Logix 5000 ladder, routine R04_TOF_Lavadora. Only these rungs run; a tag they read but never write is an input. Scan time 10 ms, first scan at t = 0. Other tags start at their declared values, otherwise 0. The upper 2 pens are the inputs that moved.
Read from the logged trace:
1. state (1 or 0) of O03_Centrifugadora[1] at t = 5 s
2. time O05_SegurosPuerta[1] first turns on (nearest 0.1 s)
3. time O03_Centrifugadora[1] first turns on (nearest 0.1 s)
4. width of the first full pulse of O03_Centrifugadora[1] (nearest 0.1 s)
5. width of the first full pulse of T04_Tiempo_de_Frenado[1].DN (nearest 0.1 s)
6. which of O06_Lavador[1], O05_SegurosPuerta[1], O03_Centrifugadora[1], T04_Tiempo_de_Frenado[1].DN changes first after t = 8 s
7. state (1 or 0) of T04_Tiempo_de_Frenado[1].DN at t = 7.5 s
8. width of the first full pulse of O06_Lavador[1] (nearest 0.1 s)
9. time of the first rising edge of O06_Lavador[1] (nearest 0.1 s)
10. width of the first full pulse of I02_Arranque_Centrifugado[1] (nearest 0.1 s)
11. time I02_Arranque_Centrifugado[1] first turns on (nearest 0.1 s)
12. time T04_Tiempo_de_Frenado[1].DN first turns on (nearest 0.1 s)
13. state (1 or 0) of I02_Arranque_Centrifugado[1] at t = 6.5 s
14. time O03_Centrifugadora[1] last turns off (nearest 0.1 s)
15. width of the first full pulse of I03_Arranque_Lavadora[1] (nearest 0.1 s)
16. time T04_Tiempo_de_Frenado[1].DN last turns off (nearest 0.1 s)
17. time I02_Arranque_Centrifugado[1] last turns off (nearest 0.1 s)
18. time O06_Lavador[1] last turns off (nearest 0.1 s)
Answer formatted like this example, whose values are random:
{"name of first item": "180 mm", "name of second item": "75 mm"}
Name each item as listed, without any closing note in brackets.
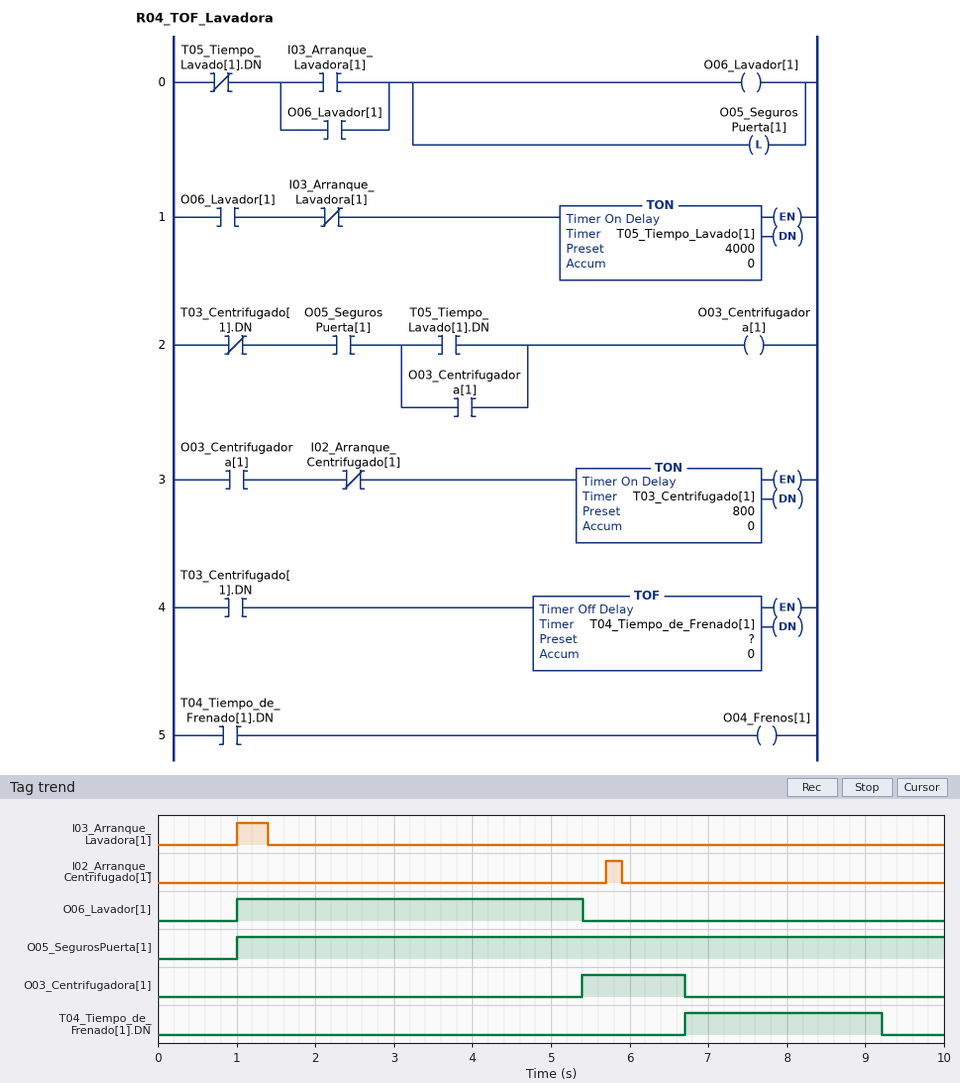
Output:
{"state (1 or 0) of O03_Centrifugadora[1] at t = 5 s": "0", "time O05_SegurosPuerta[1] first turns on": "1.0 s", "time O03_Centrifugadora[1] first turns on": "5.4 s", "width of the first full pulse of O03_Centrifugadora[1]": "1.3 s", "width of the first full pulse of T04_Tiempo_de_Frenado[1].DN": "2.5 s", "which of O06_Lavador[1], O05_SegurosPuerta[1], O03_Centrifugadora[1], T04_Tiempo_de_Frenado[1].DN changes first after t = 8 s": "T04_Tiempo_de_Frenado[1].DN", "state (1 or 0) of T04_Tiempo_de_Frenado[1].DN at t = 7.5 s": "1", "width of the first full pulse of O06_Lavador[1]": "4.4 s", "time of the first rising edge of O06_Lavador[1]": "1.0 s", "width of the first full pulse of I02_Arranque_Centrifugado[1]": "0.2 s", "time I02_Arranque_Centrifugado[1] first turns on": "5.7 s", "time T04_Tiempo_de_Frenado[1].DN first turns on": "6.7 s", "state (1 or 0) of I02_Arranque_Centrifugado[1] at t = 6.5 s": "0", "time O03_Centrifugadora[1] last turns off": "6.7 s", "width of the first full pulse of I03_Arranque_Lavadora[1]": "0.4 s", "time T04_Tiempo_de_Frenado[1].DN last turns off": "9.2 s", "time I02_Arranque_Centrifugado[1] last turns off": "5.9 s", "time O06_Lavador[1] last turns off": "5.4 s"}
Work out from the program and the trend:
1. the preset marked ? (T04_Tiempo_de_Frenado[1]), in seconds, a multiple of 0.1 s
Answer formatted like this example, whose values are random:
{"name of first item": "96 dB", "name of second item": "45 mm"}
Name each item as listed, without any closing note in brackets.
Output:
{"the preset marked ? (T04_Tiempo_de_Frenado[1]), in seconds, a multiple of 0.1 s": "2.5 s"}
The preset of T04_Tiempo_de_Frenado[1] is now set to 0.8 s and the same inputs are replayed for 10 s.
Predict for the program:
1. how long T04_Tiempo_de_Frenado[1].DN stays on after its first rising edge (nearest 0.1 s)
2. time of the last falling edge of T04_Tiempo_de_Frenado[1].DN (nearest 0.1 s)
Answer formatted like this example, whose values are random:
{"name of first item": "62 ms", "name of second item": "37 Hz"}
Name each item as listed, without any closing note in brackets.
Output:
{"how long T04_Tiempo_de_Frenado[1].DN stays on after its first rising edge": "0.8 s", "time of the last falling edge of T04_Tiempo_de_Frenado[1].DN": "7.5 s"}
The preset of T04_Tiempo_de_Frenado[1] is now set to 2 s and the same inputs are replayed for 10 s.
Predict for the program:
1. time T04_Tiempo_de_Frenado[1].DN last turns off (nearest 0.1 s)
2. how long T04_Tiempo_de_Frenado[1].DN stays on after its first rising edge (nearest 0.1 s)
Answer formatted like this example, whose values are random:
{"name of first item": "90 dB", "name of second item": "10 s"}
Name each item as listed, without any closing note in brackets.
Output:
{"time T04_Tiempo_de_Frenado[1].DN last turns off": "8.7 s", "how long T04_Tiempo_de_Frenado[1].DN stays on after its first rising edge": "2.0 s"}
